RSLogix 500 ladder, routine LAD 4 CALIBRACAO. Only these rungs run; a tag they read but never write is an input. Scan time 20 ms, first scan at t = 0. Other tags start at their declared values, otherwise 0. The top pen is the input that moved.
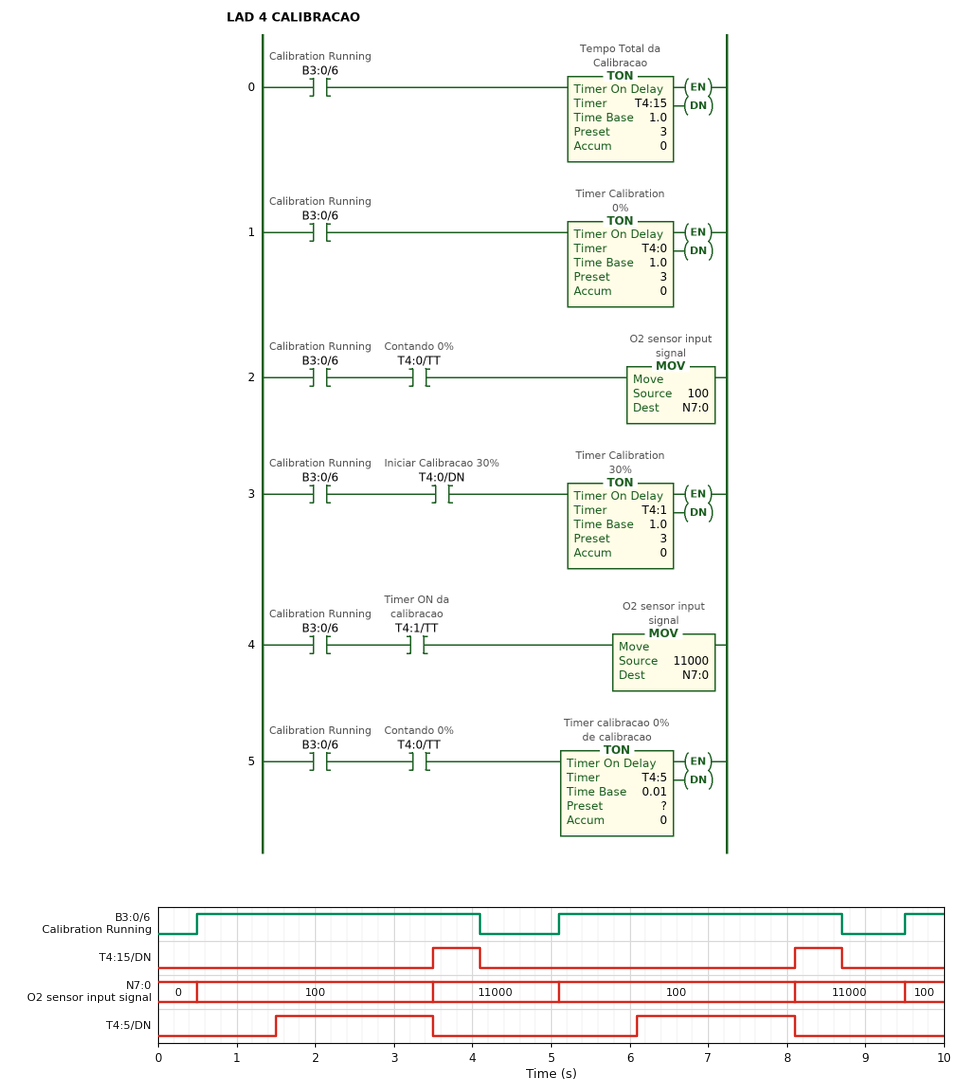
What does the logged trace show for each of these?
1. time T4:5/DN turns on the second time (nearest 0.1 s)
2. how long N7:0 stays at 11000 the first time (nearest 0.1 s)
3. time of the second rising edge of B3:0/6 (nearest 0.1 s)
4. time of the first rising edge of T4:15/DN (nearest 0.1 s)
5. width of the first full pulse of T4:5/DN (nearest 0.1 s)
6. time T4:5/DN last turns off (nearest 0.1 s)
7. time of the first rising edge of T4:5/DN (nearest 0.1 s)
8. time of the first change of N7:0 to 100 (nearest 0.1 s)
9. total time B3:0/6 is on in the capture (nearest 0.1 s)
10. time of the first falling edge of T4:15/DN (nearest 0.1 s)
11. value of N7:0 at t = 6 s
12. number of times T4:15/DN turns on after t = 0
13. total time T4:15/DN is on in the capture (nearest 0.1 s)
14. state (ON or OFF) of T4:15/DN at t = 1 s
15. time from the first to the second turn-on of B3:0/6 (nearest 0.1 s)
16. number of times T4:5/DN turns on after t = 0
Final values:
6.1 s
1.6 s
5.1 s
3.5 s
2.0 s
8.1 s
1.5 s
0.5 s
7.7 s
4.1 s
100
2
1.2 s
OFF
4.6 s
2
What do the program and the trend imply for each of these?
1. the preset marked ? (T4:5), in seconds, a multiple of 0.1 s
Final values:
1.0 s
